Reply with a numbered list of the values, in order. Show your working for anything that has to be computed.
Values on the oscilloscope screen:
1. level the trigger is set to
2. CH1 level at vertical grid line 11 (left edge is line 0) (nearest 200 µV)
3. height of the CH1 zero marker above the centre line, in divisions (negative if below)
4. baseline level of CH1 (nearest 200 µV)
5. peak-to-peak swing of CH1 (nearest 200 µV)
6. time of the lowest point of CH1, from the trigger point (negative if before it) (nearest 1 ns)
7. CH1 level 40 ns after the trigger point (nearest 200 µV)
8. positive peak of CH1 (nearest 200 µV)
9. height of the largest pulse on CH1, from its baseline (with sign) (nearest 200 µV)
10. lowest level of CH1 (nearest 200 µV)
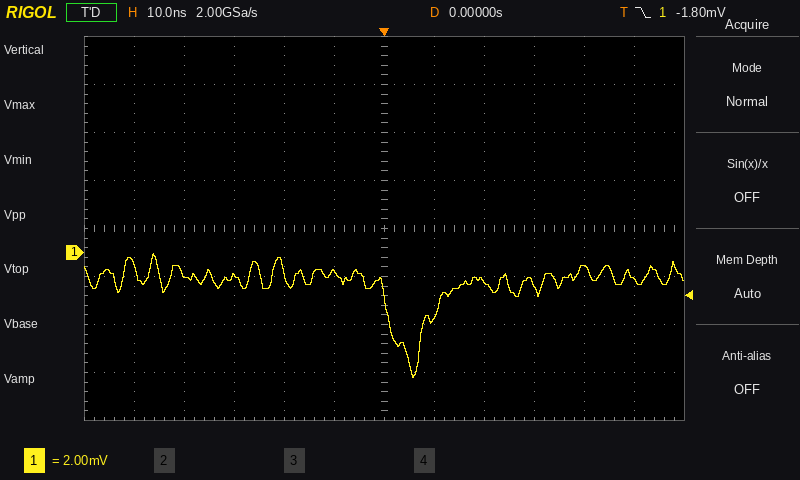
1. -1.80 mV
2. -1.2 mV
3. -0.5 div
4. -1.2 mV
5. 0.0 mV − (-5.2 mV) = 5.2 mV
6. +6 ns
7. -600 µV
8. 0.0 mV
9. -5.2 mV − (-1.2 mV) = -4.0 mV
10. -5.2 mV
